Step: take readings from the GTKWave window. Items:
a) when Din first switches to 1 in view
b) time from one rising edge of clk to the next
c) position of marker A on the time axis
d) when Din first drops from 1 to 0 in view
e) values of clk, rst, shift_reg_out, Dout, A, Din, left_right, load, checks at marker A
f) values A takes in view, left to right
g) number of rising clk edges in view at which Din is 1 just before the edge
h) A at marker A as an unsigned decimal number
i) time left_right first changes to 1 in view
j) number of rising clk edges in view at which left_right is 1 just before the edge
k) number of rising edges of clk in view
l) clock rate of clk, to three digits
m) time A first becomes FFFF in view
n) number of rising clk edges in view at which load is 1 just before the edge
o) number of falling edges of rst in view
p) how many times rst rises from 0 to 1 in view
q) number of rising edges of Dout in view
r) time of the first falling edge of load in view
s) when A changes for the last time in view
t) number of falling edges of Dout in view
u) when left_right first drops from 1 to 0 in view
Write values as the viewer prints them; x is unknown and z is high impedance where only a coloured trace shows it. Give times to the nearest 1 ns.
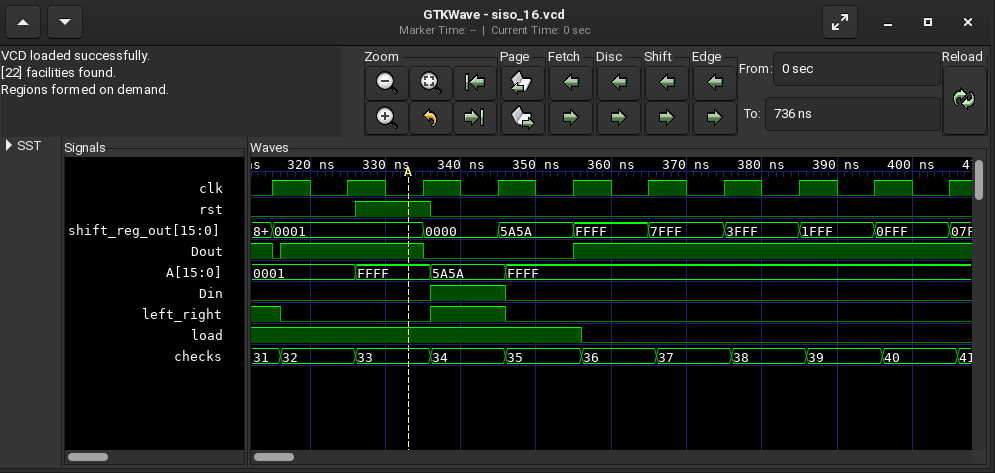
336 ns
10 ns
333 ns
346 ns
clk=0, rst=1, shift_reg_out=0001, Dout=1, A=FFFF, Din=0, left_right=0, load=1, checks=33
0001, FFFF, 5A5A, FFFF
1
65535
336 ns
2
10
100 MHz
326 ns
5
1
1
2
356 ns
346 ns
2
316 ns
